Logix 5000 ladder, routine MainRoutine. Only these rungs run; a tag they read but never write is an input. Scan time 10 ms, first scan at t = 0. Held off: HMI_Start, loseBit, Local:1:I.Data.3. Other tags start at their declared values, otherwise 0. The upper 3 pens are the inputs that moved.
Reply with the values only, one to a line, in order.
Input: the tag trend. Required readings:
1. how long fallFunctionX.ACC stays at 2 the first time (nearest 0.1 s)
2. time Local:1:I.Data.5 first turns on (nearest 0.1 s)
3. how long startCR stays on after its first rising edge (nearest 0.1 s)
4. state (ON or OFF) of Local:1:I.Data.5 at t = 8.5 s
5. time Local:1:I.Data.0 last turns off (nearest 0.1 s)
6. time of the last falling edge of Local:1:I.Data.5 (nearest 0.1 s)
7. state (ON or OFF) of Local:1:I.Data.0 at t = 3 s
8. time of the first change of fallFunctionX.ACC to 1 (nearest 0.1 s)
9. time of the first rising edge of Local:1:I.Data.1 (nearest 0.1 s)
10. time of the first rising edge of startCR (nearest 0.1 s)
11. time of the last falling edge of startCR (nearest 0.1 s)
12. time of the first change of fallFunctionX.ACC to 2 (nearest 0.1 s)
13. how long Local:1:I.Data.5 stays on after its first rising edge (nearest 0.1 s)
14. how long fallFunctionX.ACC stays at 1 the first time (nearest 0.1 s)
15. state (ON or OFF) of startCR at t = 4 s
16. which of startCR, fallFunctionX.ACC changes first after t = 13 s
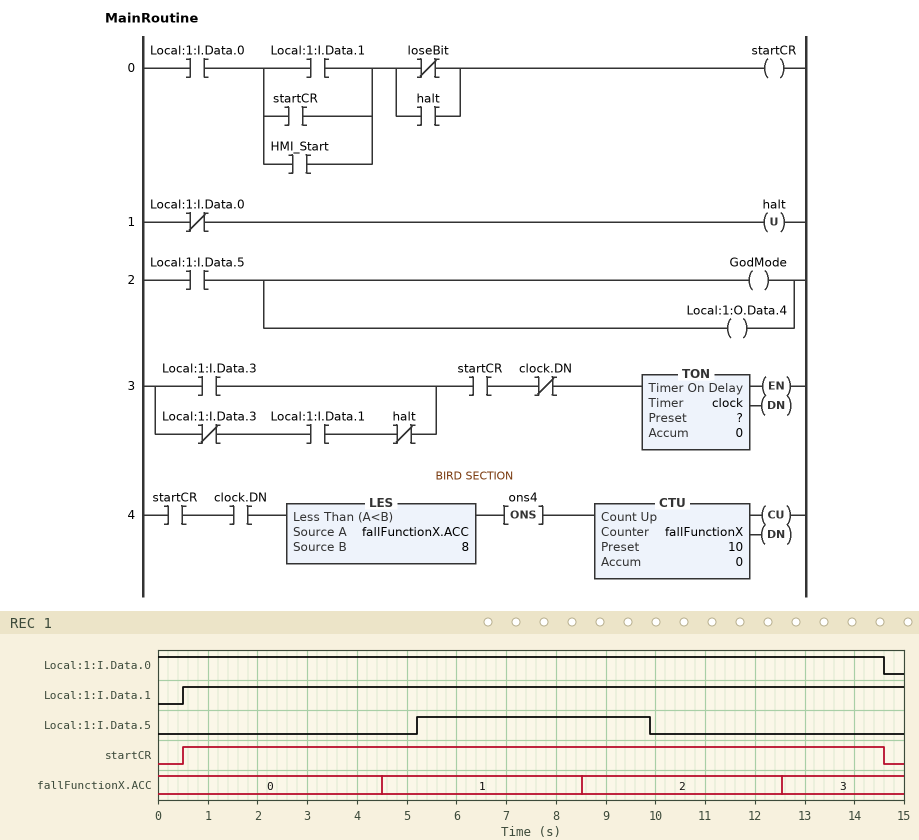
4.0 s
5.2 s
14.1 s
ON
14.6 s
9.9 s
ON
4.5 s
0.5 s
0.5 s
14.6 s
8.5 s
4.7 s
4.0 s
ON
startCR
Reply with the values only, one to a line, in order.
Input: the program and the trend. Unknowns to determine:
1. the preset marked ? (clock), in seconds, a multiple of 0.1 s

4.0 s
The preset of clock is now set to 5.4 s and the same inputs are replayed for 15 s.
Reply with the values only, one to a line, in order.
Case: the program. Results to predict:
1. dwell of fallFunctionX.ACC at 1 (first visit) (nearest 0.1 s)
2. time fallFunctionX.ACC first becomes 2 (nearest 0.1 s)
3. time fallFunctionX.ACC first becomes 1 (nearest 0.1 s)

5.4 s
11.3 s
5.9 s
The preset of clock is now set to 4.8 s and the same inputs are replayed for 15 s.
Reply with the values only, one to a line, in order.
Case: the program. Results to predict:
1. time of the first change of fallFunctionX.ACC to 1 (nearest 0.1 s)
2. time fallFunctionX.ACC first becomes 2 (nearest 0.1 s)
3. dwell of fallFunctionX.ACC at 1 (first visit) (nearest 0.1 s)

5.3 s
10.1 s
4.8 s
